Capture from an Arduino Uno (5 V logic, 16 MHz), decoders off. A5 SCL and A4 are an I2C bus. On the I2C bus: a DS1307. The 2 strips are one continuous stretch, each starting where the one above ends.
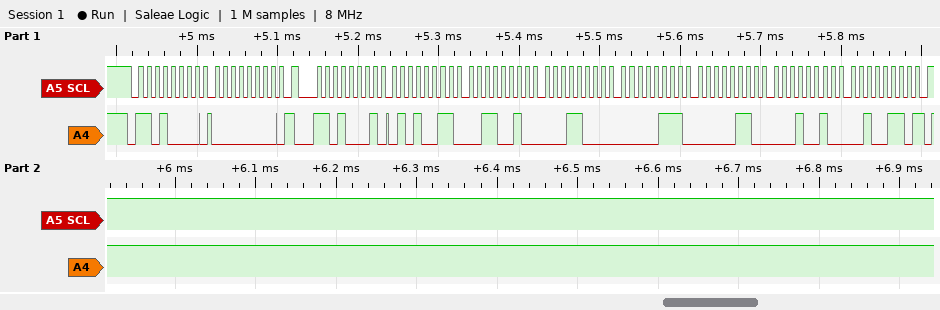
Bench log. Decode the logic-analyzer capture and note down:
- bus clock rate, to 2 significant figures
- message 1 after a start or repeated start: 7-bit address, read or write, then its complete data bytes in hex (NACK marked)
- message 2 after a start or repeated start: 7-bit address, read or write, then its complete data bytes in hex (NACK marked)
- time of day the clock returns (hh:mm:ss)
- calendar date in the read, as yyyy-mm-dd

100 kHz
0x68 write: 00
0x68 read: 53 32 18 07 06 12 26 NACK
18:32:53
2026-12-06
